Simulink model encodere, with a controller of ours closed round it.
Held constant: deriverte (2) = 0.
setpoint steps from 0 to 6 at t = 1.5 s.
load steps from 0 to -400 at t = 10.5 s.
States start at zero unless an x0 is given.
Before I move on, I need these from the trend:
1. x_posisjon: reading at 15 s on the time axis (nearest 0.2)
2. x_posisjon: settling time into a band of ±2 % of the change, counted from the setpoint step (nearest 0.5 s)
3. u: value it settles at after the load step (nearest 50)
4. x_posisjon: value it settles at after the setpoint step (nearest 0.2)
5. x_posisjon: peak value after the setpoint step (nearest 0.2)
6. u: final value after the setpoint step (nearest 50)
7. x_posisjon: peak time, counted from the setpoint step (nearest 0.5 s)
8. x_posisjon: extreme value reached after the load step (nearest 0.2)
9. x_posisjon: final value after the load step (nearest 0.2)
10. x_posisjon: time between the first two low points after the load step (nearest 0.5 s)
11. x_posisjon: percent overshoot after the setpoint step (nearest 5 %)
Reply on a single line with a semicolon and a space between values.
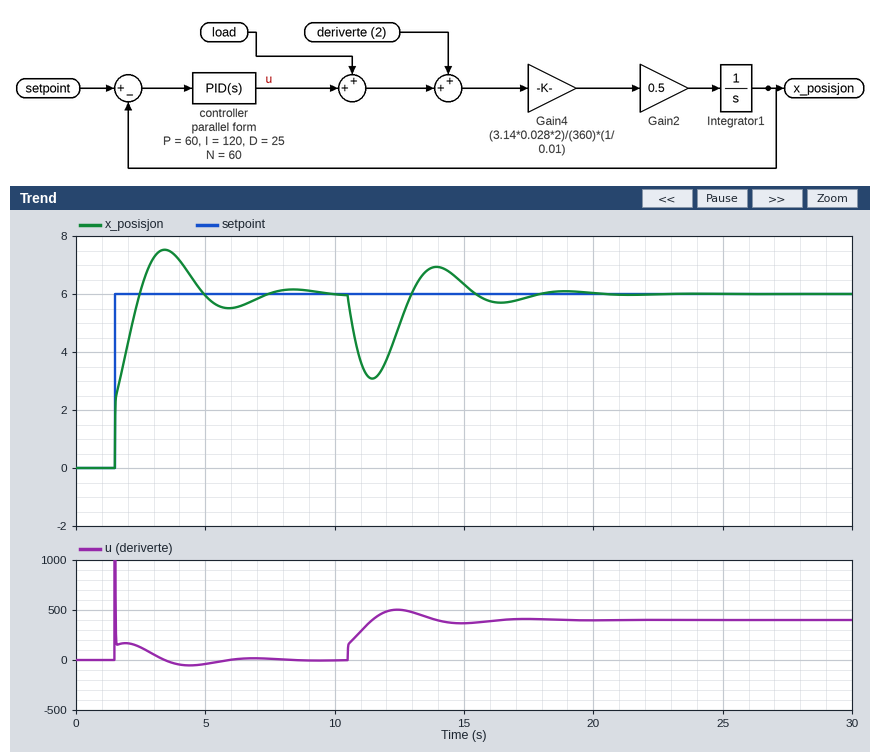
6.4; 7.5 s; 400; 6.0; 7.6; 0; 2.0 s; 3.0; 6.0; 5.0 s; 25 %
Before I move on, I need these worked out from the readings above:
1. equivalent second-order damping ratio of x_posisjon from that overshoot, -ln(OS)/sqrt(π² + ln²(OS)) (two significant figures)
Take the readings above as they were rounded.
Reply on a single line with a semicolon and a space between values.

0.40
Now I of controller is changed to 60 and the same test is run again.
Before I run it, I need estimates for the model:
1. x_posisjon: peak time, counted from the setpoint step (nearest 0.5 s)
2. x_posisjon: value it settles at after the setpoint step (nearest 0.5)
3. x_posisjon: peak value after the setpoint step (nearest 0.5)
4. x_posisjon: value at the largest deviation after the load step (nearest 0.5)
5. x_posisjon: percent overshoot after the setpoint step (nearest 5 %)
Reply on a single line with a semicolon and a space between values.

2.5 s; 6.0; 7.0; 2.5; 20 %
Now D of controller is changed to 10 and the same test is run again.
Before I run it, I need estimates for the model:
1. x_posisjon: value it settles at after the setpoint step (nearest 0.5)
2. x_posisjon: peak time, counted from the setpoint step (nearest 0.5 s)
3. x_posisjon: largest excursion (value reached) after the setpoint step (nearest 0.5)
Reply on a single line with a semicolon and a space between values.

6.0; 1.5 s; 8.0
